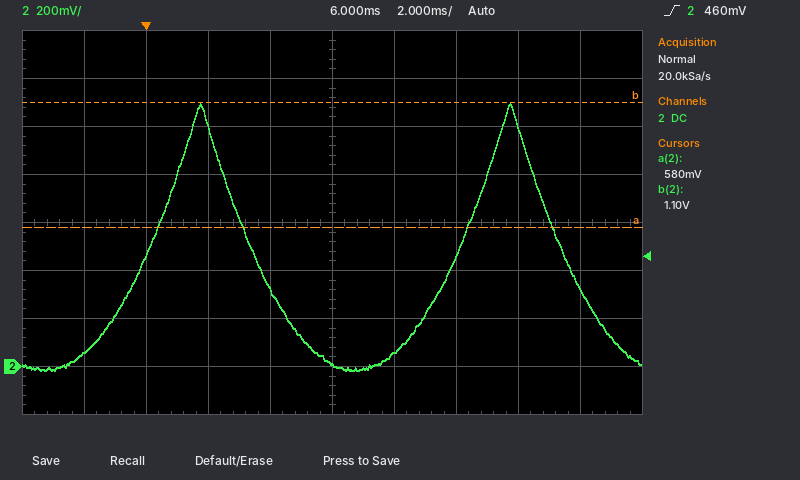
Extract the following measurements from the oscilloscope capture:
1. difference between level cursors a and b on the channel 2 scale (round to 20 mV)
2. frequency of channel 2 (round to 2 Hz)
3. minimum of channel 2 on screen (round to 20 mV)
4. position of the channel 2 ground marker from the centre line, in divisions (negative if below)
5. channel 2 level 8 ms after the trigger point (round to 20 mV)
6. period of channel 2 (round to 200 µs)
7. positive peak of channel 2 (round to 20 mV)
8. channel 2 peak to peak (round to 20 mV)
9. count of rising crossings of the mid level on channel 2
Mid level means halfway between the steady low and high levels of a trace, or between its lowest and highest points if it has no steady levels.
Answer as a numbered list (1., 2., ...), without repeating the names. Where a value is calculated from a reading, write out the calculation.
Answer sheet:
1. 520 mV
2. 1 / 10.0 ms ≈ 100 Hz
3. -20 mV
4. -3.0 div
5. 60 mV
6. 10.0 ms
7. 1.10 V
8. 1.10 V − (-20 mV) = 1.12 V
9. 2
